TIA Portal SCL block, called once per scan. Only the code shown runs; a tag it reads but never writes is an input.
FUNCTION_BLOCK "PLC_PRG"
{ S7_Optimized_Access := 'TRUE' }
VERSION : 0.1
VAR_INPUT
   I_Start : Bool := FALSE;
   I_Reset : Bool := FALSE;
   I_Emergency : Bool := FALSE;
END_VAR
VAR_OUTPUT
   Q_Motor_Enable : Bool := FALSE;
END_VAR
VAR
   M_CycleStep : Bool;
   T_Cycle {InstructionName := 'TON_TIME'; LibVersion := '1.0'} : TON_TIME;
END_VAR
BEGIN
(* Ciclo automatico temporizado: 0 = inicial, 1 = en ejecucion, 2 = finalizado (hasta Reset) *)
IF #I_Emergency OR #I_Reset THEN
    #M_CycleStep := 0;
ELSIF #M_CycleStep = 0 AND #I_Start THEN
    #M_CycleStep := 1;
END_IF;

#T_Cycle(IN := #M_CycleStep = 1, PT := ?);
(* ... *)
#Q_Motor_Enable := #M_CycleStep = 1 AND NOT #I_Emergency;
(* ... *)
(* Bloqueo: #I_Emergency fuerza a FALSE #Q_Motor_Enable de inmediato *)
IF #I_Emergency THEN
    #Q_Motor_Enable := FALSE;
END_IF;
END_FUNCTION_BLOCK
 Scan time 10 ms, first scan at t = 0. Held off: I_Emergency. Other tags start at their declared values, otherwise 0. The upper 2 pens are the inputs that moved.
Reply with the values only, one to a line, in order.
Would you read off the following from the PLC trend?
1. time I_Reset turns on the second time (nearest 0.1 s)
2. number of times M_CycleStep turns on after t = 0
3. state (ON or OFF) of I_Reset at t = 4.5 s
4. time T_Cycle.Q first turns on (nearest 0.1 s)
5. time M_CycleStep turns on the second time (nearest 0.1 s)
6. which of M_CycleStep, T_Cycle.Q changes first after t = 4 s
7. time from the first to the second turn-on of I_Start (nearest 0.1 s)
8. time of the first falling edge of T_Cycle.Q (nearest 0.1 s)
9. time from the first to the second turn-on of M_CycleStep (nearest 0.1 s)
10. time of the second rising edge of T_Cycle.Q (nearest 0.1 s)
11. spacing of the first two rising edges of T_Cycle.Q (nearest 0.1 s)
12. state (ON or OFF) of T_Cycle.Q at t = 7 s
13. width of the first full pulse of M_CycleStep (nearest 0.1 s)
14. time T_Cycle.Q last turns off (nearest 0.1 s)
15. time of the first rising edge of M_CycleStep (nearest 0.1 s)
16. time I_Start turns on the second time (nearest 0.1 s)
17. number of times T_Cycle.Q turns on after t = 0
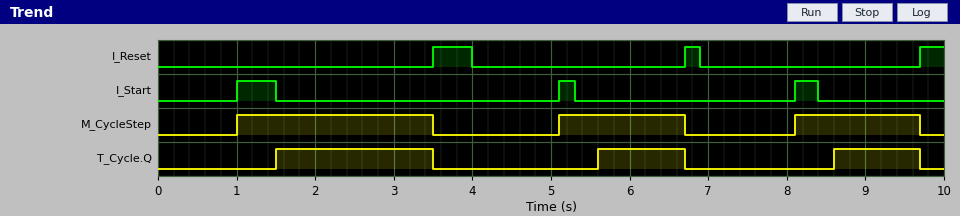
6.7 s
3
OFF
1.5 s
5.1 s
M_CycleStep
4.1 s
3.5 s
4.1 s
5.6 s
4.1 s
OFF
2.5 s
9.7 s
1.0 s
5.1 s
3
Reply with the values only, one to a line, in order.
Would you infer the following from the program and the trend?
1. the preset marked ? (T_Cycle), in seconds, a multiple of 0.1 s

0.5 s
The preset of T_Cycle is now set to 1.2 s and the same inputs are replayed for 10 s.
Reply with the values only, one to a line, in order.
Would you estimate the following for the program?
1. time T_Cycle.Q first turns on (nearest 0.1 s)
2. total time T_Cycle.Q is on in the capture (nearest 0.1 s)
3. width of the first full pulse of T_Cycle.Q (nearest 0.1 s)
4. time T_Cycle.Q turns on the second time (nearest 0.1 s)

2.2 s
2.1 s
1.3 s
6.3 s
